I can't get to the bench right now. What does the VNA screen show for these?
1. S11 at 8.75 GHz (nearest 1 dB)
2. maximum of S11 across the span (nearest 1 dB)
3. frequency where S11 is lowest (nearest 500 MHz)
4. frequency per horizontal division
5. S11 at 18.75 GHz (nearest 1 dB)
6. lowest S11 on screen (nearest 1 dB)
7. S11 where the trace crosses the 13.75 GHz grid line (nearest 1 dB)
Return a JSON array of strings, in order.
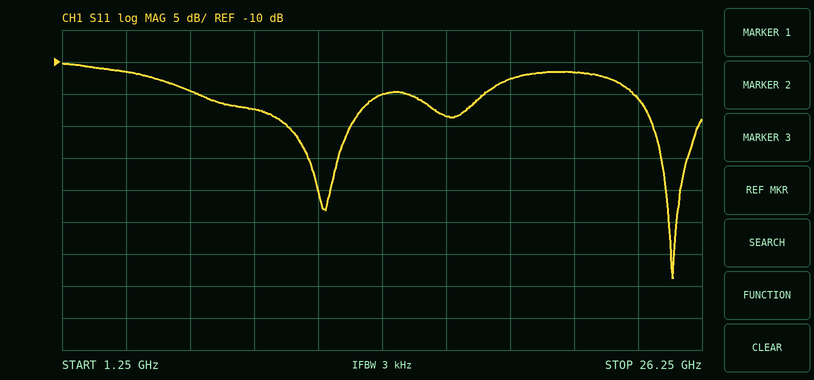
["-17 dB", "-10 dB", "25.0 GHz", "2.5 GHz", "-13 dB", "-44 dB", "-15 dB"]
